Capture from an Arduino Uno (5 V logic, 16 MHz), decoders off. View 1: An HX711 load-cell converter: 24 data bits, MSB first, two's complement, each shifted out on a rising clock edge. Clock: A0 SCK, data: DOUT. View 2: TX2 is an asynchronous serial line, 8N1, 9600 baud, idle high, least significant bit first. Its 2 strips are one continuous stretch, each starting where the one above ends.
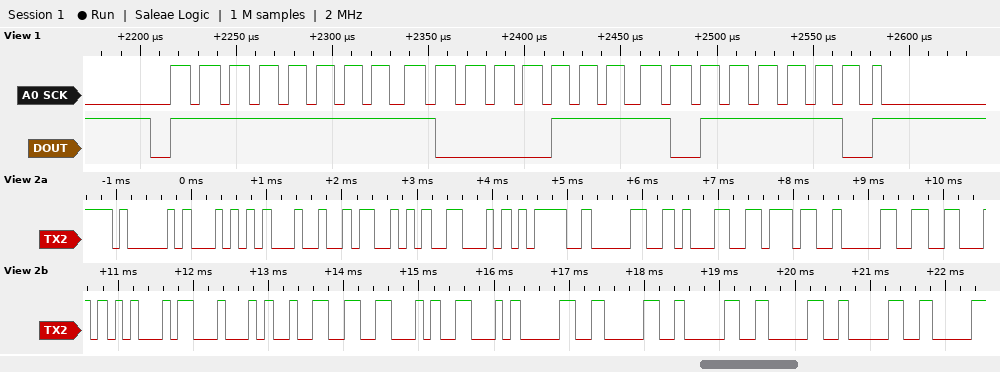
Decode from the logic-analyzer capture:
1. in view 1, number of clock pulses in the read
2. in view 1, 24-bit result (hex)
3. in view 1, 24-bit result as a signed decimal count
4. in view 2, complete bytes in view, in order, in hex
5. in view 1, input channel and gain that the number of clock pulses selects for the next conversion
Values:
25
0xFF87BE
-30786
0x41 0x54 0x24 0x53 0x46 0x3D 0x30 0x31 0x37 0x30 0x46 0x45 0x44 0x32 0x46 0x46 0x30 0x30 0x30 0x30 0x30
channel A, gain 128
